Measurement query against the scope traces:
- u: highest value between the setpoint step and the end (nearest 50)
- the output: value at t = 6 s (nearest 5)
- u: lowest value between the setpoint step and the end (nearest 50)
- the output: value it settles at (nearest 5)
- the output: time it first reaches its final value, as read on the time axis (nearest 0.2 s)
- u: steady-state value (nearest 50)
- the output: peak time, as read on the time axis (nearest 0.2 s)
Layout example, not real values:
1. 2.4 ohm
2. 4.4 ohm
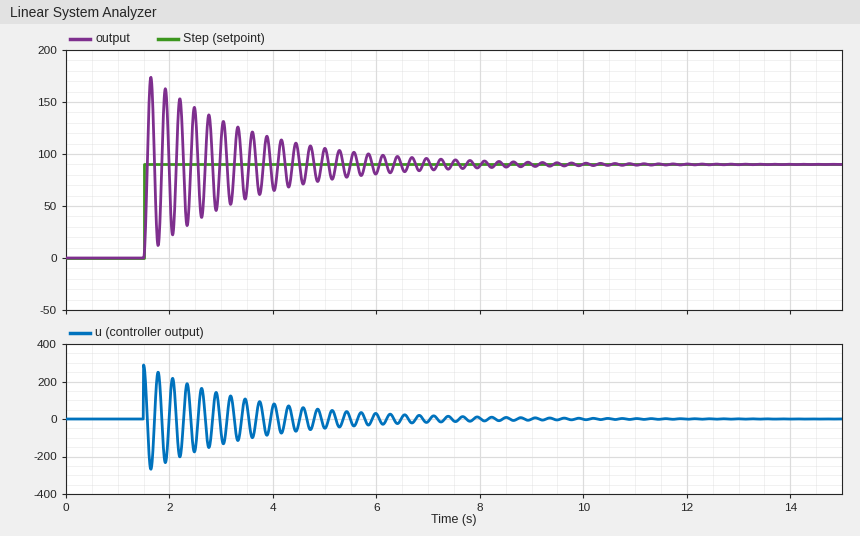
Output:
1. 300
2. 80
3. -250
4. 90
5. 1.6 s
6. 0
7. 1.6 s
